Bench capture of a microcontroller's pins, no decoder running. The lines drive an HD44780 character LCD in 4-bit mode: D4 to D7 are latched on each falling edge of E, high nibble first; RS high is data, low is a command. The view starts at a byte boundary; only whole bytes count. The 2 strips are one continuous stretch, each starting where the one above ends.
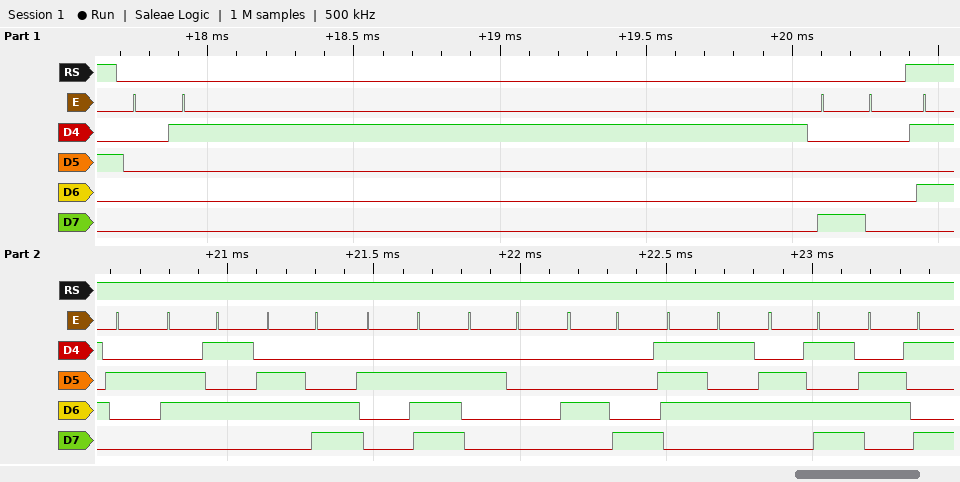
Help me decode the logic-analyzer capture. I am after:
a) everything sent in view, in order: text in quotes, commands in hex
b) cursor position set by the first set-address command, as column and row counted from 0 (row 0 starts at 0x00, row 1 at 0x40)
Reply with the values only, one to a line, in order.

0x01 0x80 "Rel. Humi"
column 0, row 0
